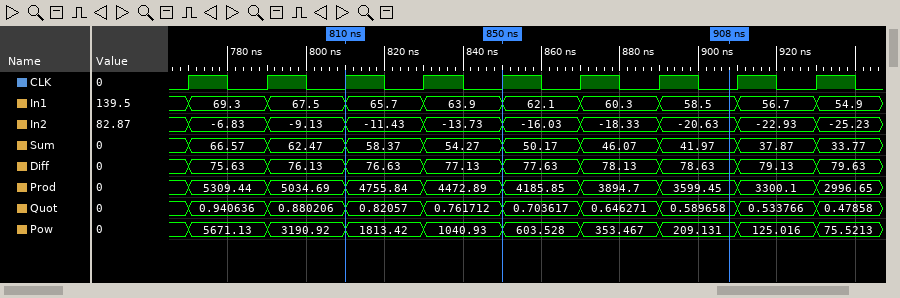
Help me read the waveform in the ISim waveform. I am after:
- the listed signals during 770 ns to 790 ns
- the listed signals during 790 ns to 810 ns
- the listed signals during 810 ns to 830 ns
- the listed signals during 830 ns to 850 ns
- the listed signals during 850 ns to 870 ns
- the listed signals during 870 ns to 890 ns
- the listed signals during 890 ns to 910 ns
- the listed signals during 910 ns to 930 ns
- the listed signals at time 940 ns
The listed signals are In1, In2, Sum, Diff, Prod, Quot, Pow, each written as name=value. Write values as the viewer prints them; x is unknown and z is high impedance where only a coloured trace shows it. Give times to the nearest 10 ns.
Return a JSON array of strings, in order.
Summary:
["In1=69.3, In2=-6.83, Sum=66.57, Diff=75.63, Prod=5309.44, Quot=0.940636, Pow=5671.13", "In1=67.5, In2=-9.13, Sum=62.47, Diff=76.13, Prod=5034.69, Quot=0.880206, Pow=3190.92", "In1=65.7, In2=-11.43, Sum=58.37, Diff=76.63, Prod=4755.84, Quot=0.82057, Pow=1813.42", "In1=63.9, In2=-13.73, Sum=54.27, Diff=77.13, Prod=4472.89, Quot=0.761712, Pow=1040.93", "In1=62.1, In2=-16.03, Sum=50.17, Diff=77.63, Prod=4185.85, Quot=0.703617, Pow=603.528", "In1=60.3, In2=-18.33, Sum=46.07, Diff=78.13, Prod=3894.7, Quot=0.646271, Pow=353.467", "In1=58.5, In2=-20.63, Sum=41.97, Diff=78.63, Prod=3599.45, Quot=0.589658, Pow=209.131", "In1=56.7, In2=-22.93, Sum=37.87, Diff=79.13, Prod=3300.1, Quot=0.533766, Pow=125.016", "In1=54.9, In2=-25.23, Sum=33.77, Diff=79.63, Prod=2996.65, Quot=0.47858, Pow=75.5213"]
